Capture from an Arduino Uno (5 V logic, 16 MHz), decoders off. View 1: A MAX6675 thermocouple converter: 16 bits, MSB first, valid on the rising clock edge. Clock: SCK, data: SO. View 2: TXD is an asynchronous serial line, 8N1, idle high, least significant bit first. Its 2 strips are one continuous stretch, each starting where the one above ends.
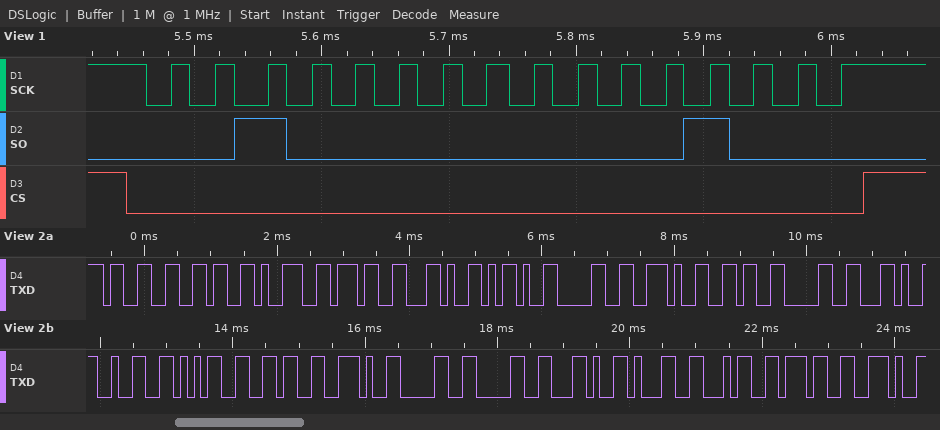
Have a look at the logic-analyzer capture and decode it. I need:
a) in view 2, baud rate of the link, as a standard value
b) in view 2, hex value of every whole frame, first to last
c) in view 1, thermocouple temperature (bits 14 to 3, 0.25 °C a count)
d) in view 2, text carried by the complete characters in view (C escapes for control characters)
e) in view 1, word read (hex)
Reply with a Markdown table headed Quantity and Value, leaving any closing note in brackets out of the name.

| Quantity | Value |
|---|---|
| in view 2, baud rate of the link, as a standard value | 9600 baud |
| in view 2, hex value of every whole frame, first to last | 33 36 39 37 2C 2D 30 2E 36 30 2C 32 35 36 2E 30 30 2C 31 34 37 2E |
| in view 1, thermocouple temperature | 256.25 °C |
| in view 2, text carried by the complete characters in view | "3697,-0.60,256.00,147." |
| in view 1, word read | 0x2008 |
